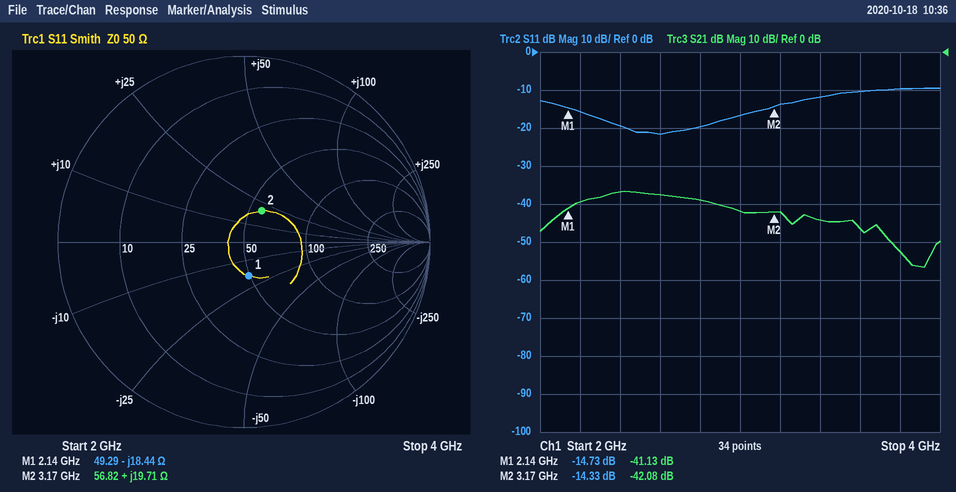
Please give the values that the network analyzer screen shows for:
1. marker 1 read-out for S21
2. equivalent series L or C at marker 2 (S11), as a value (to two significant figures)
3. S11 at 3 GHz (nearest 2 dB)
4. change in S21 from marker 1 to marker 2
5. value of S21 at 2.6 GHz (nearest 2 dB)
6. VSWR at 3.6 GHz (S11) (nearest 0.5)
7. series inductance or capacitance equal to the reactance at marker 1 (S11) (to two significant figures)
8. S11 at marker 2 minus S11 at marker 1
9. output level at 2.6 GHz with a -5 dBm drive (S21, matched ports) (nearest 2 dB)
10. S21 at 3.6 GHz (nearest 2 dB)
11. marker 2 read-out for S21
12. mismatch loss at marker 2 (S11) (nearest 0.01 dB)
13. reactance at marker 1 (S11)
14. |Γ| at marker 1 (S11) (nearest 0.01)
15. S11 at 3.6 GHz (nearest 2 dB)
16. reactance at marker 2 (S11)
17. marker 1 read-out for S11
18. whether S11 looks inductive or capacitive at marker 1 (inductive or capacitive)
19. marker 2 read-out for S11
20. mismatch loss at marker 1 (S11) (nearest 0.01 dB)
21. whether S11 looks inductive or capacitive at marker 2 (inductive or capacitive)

-41.13 dB
990 pH
-16 dB
-0.95 dB
-38 dB
2.0
4.0 pF
0.40 dB
-42 dBm
-46 dB
-42.08 dB
0.16 dB
-18.44 Ω
0.18
-10 dB
+19.71 Ω
-14.73 dB
capacitive
-14.33 dB
0.15 dB
inductive
